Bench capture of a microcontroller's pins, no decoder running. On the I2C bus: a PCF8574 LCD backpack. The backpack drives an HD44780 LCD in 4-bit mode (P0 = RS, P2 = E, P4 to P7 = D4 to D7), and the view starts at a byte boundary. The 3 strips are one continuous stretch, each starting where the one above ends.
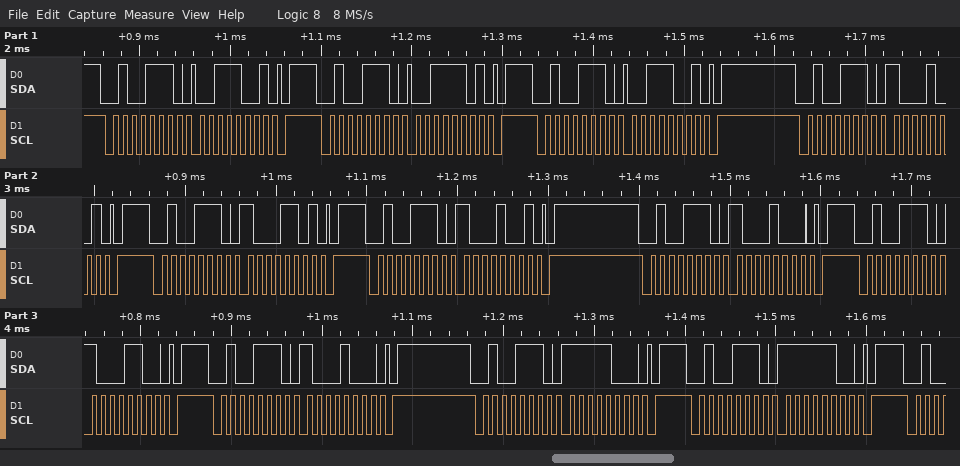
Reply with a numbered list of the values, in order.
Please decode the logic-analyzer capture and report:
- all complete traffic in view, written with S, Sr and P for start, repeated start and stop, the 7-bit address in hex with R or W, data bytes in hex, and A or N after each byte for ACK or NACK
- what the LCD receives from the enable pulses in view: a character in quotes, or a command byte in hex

1. S 27W A 39 A P S 27W A 3D A P S 27W A 39 A P S 27W A 89 A P S 27W A 8D A P S 27W A 89 A P S 27W A 88 A P S 27W A 8C A P S 27W A 88 A P S 27W A F8 A P S 27W A FC A P
2. '8'
